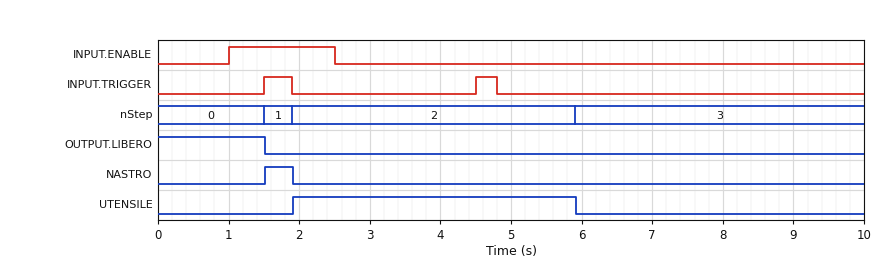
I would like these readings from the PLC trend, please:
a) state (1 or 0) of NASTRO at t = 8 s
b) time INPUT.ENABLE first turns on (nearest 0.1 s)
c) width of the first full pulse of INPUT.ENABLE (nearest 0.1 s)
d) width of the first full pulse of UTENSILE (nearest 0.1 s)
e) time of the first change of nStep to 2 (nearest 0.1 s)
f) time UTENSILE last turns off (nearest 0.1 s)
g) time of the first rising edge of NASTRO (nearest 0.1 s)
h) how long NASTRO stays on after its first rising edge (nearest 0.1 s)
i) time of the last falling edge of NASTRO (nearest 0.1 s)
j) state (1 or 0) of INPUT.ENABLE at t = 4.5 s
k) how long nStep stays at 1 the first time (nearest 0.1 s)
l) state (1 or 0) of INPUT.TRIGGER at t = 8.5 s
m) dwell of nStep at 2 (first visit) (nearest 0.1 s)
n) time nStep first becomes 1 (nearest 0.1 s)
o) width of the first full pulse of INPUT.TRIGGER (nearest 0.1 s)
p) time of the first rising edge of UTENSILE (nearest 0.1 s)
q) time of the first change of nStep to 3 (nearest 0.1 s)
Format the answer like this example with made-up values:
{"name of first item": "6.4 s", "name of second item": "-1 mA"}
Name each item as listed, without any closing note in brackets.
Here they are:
{"state (1 or 0) of NASTRO at t = 8 s": "0", "time INPUT.ENABLE first turns on": "1.0 s", "width of the first full pulse of INPUT.ENABLE": "1.5 s", "width of the first full pulse of UTENSILE": "4.0 s", "time of the first change of nStep to 2": "1.9 s", "time UTENSILE last turns off": "5.9 s", "time of the first rising edge of NASTRO": "1.5 s", "how long NASTRO stays on after its first rising edge": "0.4 s", "time of the last falling edge of NASTRO": "1.9 s", "state (1 or 0) of INPUT.ENABLE at t = 4.5 s": "0", "how long nStep stays at 1 the first time": "0.4 s", "state (1 or 0) of INPUT.TRIGGER at t = 8.5 s": "0", "dwell of nStep at 2 (first visit)": "4.0 s", "time nStep first becomes 1": "1.5 s", "width of the first full pulse of INPUT.TRIGGER": "0.4 s", "time of the first rising edge of UTENSILE": "1.9 s", "time of the first change of nStep to 3": "5.9 s"}
